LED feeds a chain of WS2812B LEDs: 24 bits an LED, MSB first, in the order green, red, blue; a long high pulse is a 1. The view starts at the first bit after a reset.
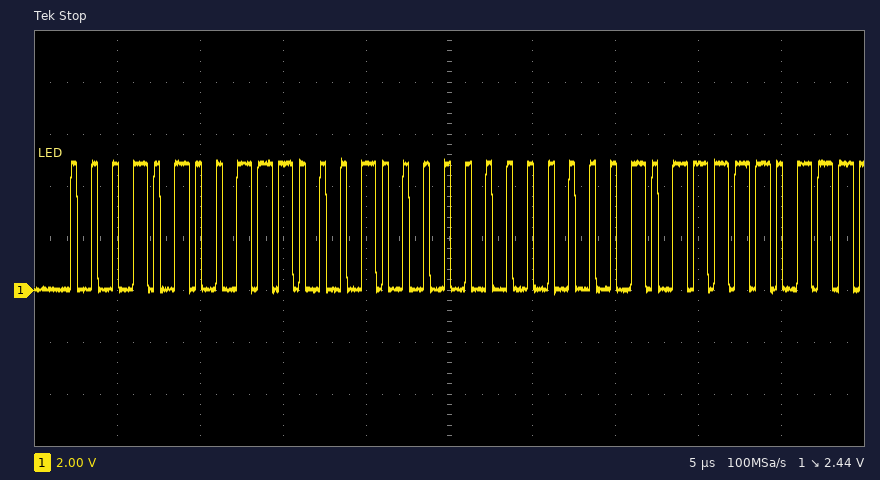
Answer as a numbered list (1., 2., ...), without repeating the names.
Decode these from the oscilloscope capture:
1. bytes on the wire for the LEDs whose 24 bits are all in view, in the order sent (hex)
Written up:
1. 14 E2 00
